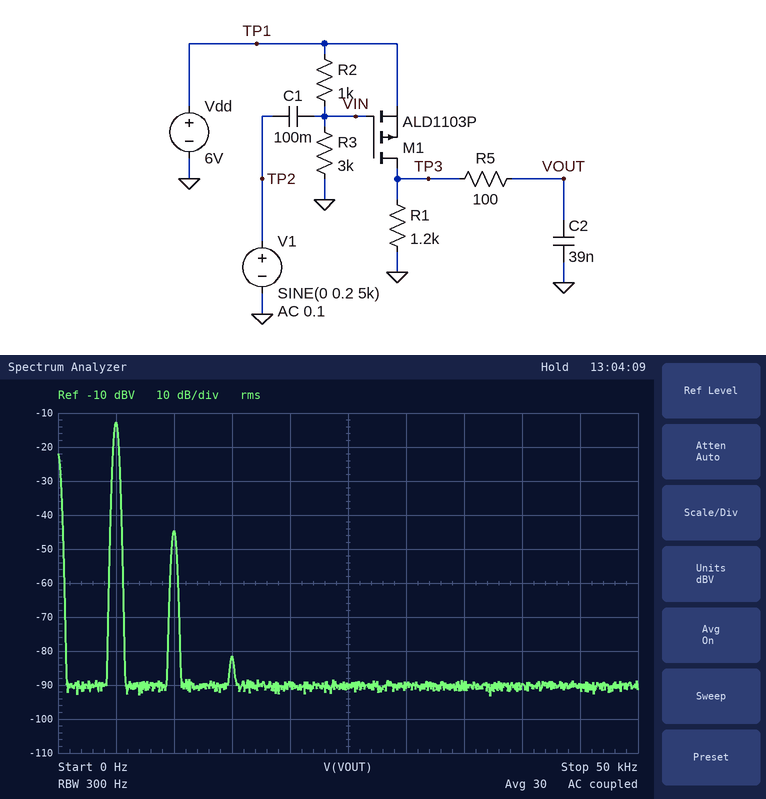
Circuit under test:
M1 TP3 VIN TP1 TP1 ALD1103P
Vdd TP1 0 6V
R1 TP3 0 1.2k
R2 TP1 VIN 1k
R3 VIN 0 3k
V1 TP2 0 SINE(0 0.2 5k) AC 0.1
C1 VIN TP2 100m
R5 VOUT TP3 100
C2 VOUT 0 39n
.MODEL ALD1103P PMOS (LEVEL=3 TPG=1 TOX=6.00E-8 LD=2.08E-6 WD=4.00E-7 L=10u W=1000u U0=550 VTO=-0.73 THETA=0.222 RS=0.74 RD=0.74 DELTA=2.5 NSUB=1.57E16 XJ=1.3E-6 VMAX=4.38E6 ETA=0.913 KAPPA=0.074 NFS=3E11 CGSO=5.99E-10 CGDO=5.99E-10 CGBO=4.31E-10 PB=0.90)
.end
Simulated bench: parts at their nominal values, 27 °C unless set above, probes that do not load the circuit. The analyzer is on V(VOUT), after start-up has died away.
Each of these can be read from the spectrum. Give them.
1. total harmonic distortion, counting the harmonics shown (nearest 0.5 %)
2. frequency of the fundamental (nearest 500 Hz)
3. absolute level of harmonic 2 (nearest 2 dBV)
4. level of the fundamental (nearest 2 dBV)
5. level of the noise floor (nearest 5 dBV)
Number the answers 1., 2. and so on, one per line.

1. 2.5 %
2. 5.0 kHz
3. -44 dBV
4. -12 dBV
5. -90 dBV
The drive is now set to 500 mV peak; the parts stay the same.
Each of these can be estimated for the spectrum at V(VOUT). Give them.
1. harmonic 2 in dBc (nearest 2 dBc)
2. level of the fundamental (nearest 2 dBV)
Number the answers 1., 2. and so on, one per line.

1. -24 dBc
2. -4 dBV
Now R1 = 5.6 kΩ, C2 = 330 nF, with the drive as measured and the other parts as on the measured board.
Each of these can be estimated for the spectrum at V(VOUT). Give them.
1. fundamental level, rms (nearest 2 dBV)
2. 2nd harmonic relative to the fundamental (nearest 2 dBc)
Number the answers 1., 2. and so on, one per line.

1. -34 dBV
2. -28 dBc
